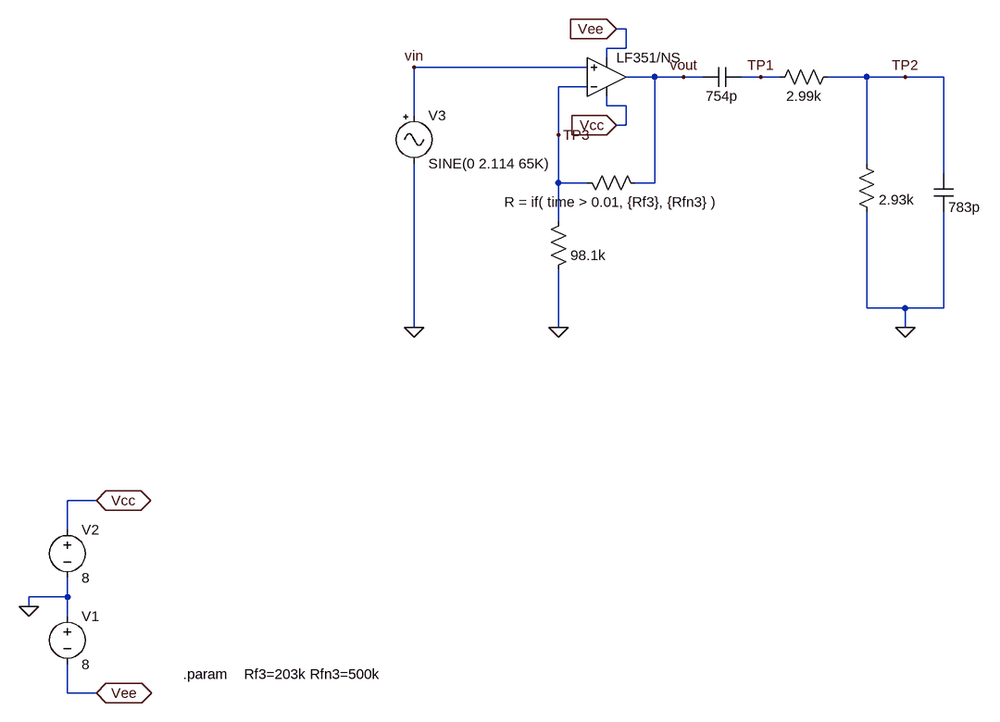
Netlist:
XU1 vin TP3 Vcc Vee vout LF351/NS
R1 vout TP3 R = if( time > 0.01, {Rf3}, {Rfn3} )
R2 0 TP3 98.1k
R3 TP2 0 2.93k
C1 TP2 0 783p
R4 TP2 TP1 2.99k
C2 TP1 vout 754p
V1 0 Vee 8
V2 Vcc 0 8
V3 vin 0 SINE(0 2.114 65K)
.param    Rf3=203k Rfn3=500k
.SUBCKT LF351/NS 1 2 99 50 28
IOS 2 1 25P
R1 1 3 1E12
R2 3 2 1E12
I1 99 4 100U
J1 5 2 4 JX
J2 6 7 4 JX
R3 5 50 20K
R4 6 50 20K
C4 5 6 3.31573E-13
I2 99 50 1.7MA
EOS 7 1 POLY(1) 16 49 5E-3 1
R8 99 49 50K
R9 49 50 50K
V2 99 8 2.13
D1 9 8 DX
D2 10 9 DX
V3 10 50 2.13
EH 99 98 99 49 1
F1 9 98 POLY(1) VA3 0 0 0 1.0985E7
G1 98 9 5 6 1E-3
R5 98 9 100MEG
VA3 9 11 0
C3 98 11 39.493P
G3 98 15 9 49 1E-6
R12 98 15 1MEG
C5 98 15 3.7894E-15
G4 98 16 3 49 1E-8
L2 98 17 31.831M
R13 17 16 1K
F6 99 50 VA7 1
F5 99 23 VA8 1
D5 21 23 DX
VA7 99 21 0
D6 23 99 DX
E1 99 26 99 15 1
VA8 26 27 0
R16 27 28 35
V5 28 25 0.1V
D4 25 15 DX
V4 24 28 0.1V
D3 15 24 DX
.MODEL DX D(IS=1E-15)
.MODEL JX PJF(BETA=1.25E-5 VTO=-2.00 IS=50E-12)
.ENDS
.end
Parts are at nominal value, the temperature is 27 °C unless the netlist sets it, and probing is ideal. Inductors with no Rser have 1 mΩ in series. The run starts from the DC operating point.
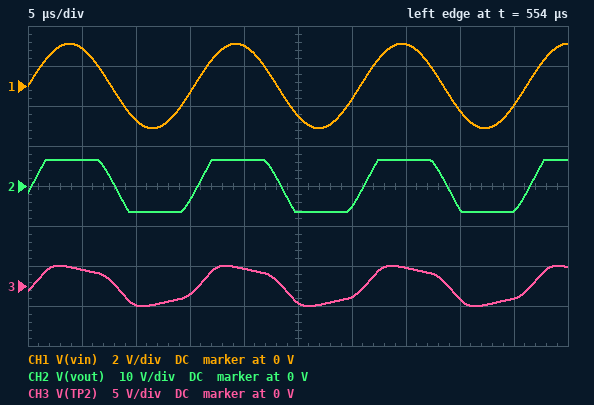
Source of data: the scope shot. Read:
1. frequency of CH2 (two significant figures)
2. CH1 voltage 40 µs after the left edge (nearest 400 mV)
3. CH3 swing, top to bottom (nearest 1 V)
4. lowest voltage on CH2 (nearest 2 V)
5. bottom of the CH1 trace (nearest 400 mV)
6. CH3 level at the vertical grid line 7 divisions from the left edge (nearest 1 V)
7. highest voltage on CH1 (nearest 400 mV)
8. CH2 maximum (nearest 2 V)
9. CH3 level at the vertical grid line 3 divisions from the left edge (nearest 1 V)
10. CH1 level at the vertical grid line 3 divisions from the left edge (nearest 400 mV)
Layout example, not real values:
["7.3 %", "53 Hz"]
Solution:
["65 kHz", "-1.2 V", "5 V", "-6 V", "-2.0 V", "2 V", "2.0 V", "6 V", "-1 V", "-400 mV"]
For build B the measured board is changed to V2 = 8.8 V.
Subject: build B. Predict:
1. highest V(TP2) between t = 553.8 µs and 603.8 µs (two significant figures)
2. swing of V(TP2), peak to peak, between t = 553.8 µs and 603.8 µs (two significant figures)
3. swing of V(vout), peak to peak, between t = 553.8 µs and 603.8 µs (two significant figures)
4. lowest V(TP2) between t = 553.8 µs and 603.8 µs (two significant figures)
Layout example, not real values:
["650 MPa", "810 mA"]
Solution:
["2.7 V", "5.3 V", "14 V", "-2.6 V"]
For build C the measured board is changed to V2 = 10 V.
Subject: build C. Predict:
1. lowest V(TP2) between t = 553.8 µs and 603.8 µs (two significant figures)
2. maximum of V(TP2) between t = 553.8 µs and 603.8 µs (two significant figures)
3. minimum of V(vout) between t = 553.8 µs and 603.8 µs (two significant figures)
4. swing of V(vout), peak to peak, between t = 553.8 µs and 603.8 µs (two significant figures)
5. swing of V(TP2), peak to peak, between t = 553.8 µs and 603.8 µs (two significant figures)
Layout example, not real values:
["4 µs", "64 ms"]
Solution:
["-2.8 V", "2.9 V", "-6.6 V", "15 V", "5.7 V"]
